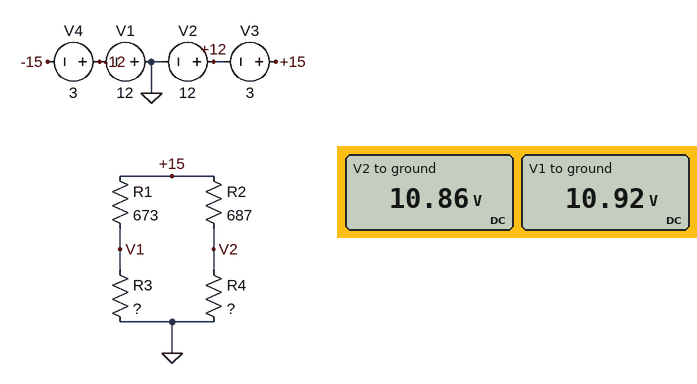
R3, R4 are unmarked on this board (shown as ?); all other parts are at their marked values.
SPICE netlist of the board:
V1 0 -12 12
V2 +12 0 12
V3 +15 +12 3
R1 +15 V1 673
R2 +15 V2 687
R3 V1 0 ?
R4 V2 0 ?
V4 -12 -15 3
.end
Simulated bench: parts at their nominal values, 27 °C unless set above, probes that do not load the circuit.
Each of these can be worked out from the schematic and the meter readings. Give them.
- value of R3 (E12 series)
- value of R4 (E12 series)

1.8 kΩ
1.8 kΩ
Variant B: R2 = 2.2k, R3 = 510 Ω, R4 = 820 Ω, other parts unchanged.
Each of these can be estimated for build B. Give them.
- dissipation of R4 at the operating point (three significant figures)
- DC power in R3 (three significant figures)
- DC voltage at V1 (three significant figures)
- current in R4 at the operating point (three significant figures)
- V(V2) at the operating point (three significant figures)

20.2 mW
82.0 mW
6.47 V
4.97 mA
4.07 V
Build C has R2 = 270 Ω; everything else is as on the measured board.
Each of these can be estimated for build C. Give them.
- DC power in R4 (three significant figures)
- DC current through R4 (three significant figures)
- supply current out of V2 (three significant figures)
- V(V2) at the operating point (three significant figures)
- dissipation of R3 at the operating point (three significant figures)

94.5 mW
7.25 mA
13.3 mA
13.0 V
66.2 mW
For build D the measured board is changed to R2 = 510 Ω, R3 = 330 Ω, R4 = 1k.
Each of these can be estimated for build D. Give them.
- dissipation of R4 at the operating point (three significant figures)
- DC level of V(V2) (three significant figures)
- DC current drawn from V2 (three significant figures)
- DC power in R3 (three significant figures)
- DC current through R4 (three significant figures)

98.7 mW
9.93 V
24.9 mA
73.8 mW
9.93 mA
